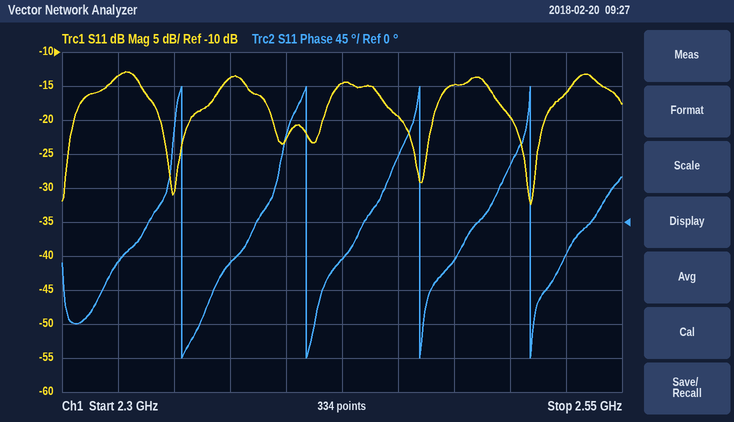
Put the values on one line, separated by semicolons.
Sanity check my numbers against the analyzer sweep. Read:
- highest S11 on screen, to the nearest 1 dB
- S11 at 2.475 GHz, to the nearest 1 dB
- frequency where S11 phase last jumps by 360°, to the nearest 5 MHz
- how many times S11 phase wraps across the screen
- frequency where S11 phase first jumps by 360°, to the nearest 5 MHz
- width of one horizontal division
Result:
-13 dB; -15 dB; 2.510 GHz; 4; 2.355 GHz; 25 MHz
